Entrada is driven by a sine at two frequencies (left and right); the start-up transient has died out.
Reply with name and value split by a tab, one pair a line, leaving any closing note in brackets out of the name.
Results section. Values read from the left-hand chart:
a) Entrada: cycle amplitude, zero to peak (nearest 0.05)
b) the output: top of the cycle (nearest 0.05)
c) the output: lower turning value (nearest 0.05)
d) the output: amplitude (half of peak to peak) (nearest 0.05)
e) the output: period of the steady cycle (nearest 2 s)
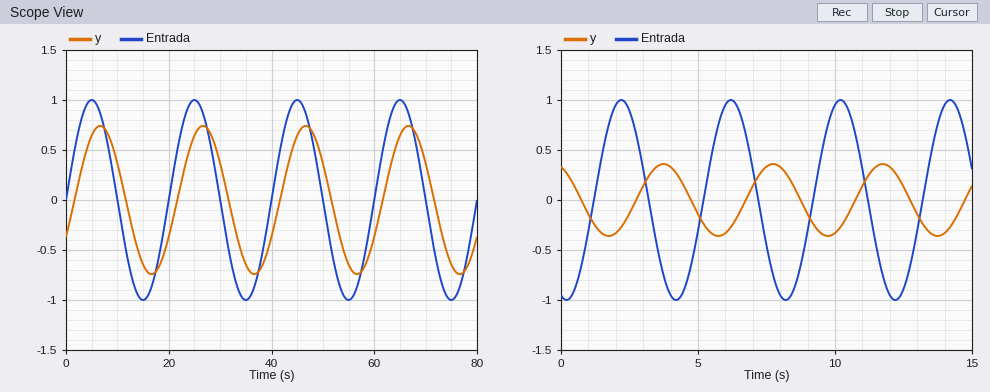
Entrada: cycle amplitude, zero to peak	1.00
the output: top of the cycle	0.75
the output: lower turning value	-0.75
the output: amplitude (half of peak to peak)	0.75
the output: period of the steady cycle	20 s
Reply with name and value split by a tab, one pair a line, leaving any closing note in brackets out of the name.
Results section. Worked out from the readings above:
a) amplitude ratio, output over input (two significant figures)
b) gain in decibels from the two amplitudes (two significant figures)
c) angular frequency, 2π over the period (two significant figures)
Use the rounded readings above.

amplitude ratio, output over input	0.75
gain in decibels from the two amplitudes	-2.5 dB
angular frequency, 2π over the period	0.31 rad/s
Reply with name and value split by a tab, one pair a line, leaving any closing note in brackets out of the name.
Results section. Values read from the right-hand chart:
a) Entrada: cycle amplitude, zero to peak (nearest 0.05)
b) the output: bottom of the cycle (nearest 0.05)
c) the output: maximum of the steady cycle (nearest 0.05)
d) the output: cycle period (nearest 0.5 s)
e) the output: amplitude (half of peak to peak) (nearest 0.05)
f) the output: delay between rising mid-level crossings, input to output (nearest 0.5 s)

Entrada: cycle amplitude, zero to peak	1.00
the output: bottom of the cycle	-0.35
the output: maximum of the steady cycle	0.35
the output: cycle period	4.0 s
the output: amplitude (half of peak to peak)	0.35
the output: delay between rising mid-level crossings, input to output	1.5 s
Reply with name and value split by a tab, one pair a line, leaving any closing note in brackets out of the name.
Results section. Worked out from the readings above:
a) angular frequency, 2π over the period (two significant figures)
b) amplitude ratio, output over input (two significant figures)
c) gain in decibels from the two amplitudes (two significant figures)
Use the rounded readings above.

angular frequency, 2π over the period	1.6 rad/s
amplitude ratio, output over input	0.35
gain in decibels from the two amplitudes	-9.1 dB
